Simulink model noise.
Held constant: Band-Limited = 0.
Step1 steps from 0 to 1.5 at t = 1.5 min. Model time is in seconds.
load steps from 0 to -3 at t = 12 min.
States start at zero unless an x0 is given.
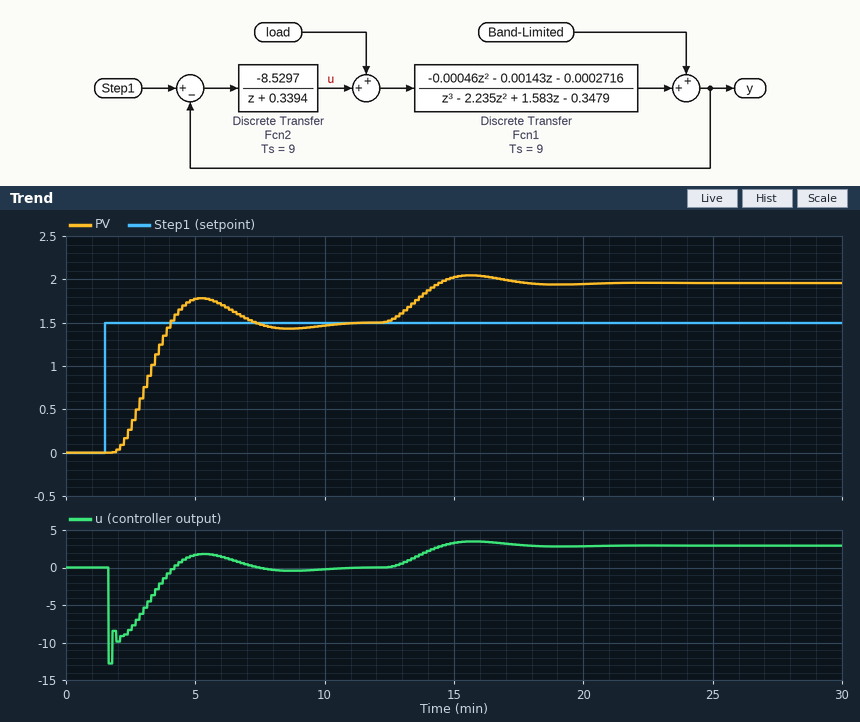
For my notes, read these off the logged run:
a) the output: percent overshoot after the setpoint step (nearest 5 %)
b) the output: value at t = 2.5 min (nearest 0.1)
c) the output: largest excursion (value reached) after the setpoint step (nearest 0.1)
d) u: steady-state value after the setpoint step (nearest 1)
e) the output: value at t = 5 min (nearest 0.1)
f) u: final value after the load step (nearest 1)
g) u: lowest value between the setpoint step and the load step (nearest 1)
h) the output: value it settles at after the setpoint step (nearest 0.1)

20 %
0.3
1.8
0
1.8
3
-13
1.5
